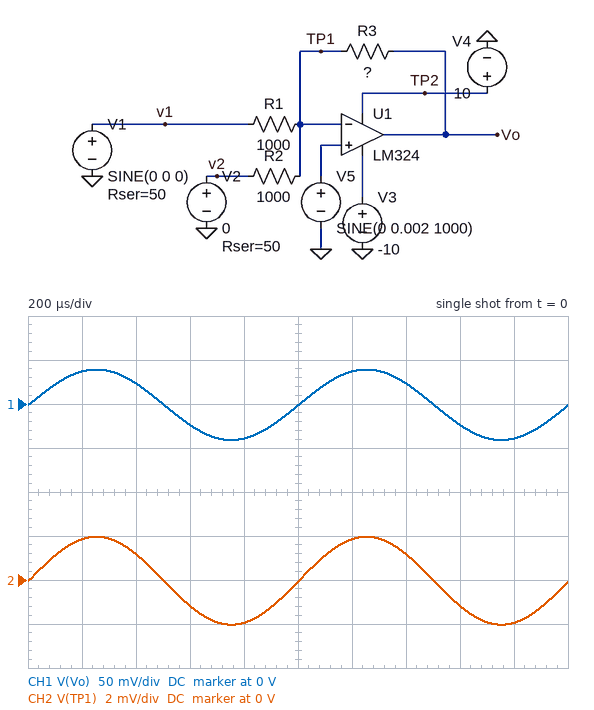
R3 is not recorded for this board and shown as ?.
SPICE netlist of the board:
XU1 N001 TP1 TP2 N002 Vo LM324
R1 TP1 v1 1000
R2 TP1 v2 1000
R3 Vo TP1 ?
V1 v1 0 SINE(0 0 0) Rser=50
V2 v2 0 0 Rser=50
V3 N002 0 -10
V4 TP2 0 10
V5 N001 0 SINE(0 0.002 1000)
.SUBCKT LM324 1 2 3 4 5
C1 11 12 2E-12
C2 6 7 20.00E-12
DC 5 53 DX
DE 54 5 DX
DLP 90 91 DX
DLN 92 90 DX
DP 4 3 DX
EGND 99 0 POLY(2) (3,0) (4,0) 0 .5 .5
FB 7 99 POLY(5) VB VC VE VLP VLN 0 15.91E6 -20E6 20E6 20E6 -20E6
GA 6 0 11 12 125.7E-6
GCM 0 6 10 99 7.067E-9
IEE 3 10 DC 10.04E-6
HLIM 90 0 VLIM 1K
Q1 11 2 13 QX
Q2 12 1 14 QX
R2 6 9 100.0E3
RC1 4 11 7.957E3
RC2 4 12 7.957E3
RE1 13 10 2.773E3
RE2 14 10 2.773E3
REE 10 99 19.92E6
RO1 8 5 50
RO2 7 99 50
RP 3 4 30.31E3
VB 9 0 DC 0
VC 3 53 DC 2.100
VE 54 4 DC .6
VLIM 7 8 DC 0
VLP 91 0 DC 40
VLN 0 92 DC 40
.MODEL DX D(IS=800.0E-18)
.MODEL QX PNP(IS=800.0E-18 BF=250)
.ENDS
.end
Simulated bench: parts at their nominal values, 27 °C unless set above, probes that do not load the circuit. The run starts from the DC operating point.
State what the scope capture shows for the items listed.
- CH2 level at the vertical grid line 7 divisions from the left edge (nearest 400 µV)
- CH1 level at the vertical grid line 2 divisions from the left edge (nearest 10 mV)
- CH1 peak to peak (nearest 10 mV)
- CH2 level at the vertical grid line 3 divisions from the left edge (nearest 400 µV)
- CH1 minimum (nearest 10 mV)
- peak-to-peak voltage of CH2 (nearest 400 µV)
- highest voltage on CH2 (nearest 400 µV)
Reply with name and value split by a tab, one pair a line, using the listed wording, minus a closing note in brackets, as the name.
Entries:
CH2 level at the vertical grid line 7 divisions from the left edge	1.2 mV
CH1 level at the vertical grid line 2 divisions from the left edge	20 mV
CH1 peak to peak	80 mV
CH2 level at the vertical grid line 3 divisions from the left edge	-1.2 mV
CH1 minimum	-40 mV
peak-to-peak voltage of CH2	4.0 mV
highest voltage on CH2	2.0 mV
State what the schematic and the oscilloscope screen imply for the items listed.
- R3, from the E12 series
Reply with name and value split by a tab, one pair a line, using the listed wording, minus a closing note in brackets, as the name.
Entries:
R3, from the E12 series	10 kΩ
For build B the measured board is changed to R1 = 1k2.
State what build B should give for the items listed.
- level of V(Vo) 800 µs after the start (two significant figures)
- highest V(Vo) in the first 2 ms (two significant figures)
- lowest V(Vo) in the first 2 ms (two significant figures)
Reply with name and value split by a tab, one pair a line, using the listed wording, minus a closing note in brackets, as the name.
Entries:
level of V(Vo) 800 µs after the start	-36 mV
highest V(Vo) in the first 2 ms	36 mV
lowest V(Vo) in the first 2 ms	-38 mV
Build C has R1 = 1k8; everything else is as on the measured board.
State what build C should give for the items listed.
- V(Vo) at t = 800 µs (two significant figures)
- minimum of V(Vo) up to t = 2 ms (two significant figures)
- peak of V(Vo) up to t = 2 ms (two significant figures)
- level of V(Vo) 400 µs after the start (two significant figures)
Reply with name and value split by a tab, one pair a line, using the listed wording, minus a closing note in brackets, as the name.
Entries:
V(Vo) at t = 800 µs	-31 mV
minimum of V(Vo) up to t = 2 ms	-33 mV
peak of V(Vo) up to t = 2 ms	31 mV
level of V(Vo) 400 µs after the start	18 mV
